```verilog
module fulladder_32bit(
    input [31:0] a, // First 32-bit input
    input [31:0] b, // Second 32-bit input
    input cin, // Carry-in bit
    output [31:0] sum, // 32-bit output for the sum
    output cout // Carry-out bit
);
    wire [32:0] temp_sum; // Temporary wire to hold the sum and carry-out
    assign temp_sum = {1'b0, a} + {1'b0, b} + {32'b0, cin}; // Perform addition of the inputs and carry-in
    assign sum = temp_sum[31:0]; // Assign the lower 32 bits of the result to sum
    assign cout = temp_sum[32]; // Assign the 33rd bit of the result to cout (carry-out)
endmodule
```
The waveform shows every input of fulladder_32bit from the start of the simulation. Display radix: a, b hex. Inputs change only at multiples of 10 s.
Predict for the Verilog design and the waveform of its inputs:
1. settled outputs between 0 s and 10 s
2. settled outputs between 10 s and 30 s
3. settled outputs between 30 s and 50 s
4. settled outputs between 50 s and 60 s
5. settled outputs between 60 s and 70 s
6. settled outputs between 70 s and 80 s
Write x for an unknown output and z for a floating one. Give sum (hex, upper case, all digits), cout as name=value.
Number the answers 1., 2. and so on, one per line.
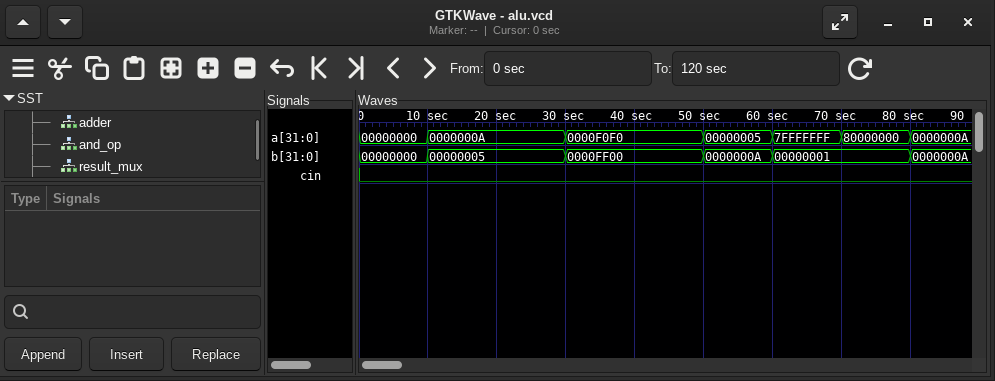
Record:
1. sum=00000000, cout=0
2. sum=0000000F, cout=0
3. sum=0001EFF0, cout=0
4. sum=0000000F, cout=0
5. sum=80000000, cout=0
6. sum=80000001, cout=0
